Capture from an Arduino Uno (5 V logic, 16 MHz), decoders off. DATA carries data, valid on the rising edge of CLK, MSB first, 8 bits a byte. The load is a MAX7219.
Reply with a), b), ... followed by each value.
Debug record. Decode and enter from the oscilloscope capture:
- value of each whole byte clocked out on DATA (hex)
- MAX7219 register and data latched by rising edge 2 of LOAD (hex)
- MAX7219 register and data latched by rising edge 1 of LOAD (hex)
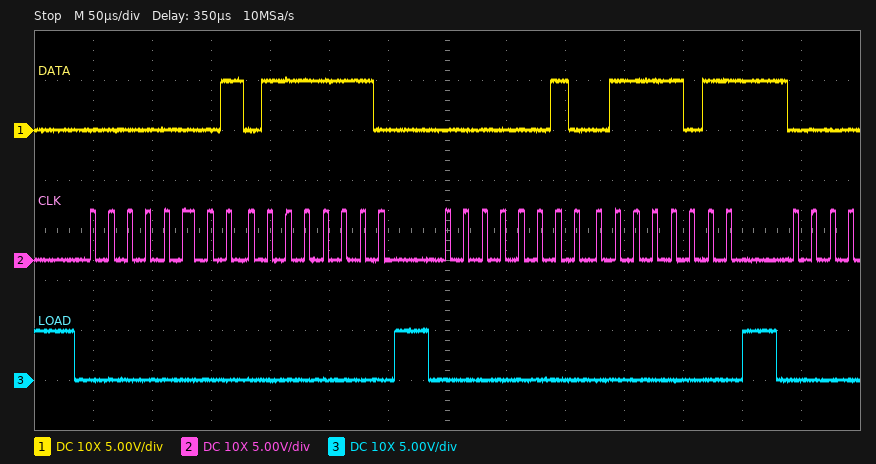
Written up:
a) 01 7E 02 7B
b) register 0x2, data 0x7B
c) register 0x1, data 0x7E
